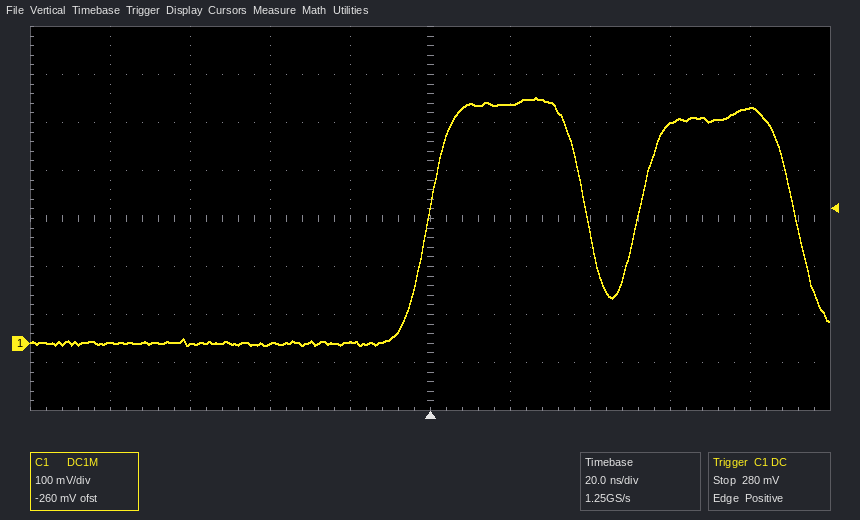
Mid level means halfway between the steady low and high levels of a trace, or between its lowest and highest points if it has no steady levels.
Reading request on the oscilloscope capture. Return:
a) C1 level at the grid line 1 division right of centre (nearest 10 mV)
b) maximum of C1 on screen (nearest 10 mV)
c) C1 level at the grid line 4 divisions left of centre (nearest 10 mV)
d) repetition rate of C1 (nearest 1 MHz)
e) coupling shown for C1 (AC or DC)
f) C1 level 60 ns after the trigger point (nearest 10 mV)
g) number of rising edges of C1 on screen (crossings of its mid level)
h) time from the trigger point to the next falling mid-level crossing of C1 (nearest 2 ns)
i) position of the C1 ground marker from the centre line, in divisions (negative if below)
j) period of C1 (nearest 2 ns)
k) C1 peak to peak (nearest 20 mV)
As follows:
500 mV
510 mV
0 mV
19 MHz
DC
460 mV
2
40 ns
-2.6 div
52 ns
520 mV
